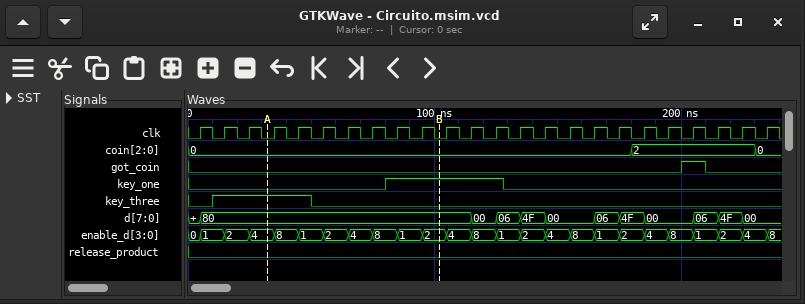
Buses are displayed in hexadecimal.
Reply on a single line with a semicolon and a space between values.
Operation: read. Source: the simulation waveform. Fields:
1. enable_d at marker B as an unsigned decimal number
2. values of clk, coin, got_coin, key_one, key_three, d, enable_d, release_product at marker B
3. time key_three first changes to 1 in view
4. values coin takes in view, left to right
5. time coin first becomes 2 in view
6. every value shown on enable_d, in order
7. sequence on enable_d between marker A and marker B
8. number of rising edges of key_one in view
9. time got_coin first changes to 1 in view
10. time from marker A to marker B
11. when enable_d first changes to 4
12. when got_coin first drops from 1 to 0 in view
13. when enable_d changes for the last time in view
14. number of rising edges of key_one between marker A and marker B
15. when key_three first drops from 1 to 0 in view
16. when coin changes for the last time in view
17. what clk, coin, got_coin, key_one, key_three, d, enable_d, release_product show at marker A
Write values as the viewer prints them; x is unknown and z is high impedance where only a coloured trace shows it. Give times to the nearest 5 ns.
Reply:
2; clk=0, coin=0, got_coin=0, key_one=1, key_three=0, d=80, enable_d=2, release_product=0; 10 ns; 0, 2, 0; 180 ns; 0, 1, 2, 4, 8, 1, 2, 4, 8, 1, 2, 4, 8, 1, 2, 4, 8, 1, 2, 4, 8, 1, 2, 4, 8; 4, 8, 1, 2, 4, 8, 1, 2; 1; 200 ns; 70 ns; 25 ns; 210 ns; 235 ns; 1; 50 ns; 230 ns; clk=0, coin=0, got_coin=0, key_one=0, key_three=1, d=80, enable_d=4, release_product=0
